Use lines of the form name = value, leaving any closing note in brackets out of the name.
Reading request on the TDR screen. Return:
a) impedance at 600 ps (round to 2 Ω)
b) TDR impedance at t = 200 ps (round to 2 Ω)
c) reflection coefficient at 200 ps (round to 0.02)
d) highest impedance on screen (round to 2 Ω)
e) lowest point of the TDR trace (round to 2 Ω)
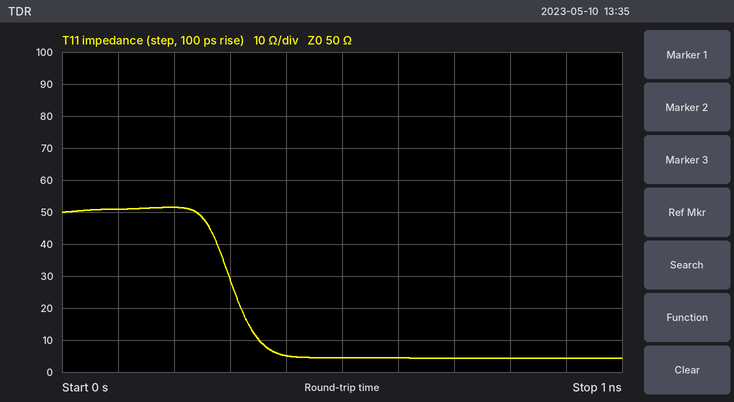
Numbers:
impedance at 600 ps = 4 Ω
TDR impedance at t = 200 ps = 52 Ω
reflection coefficient at 200 ps = +0.02
highest impedance on screen = 52 Ω
lowest point of the TDR trace = 4 Ω
